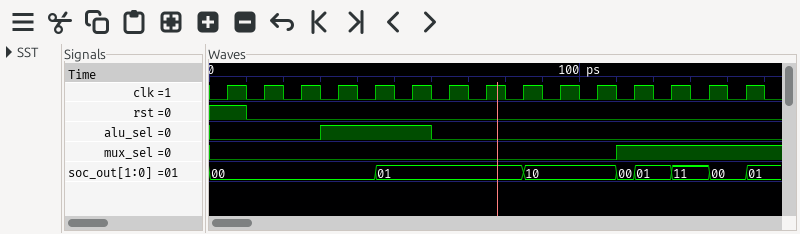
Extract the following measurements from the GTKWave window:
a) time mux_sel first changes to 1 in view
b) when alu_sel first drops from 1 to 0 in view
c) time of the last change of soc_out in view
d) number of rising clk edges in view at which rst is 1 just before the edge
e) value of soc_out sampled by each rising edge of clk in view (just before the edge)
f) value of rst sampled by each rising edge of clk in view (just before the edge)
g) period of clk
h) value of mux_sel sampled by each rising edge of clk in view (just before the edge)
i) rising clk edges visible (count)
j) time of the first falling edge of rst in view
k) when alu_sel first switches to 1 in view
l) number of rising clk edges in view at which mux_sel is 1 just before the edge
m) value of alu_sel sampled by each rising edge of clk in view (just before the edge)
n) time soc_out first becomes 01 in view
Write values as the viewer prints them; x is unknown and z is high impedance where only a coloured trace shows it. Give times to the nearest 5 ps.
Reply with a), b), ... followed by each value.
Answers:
a) 110 ps
b) 60 ps
c) 145 ps
d) 1
e) 00, 00, 00, 00, 00, 01, 01, 01, 01, 10, 10, 00, 01, 11, 00
f) 1 0 0 0 0 0 0 0 0 0 0 0 0 0 0
g) 10 ps
h) 0 0 0 0 0 0 0 0 0 0 0 1 1 1 1
i) 15
j) 10 ps
k) 30 ps
l) 4
m) 0 0 0 1 1 1 0 0 0 0 0 0 0 0 0
n) 45 ps
